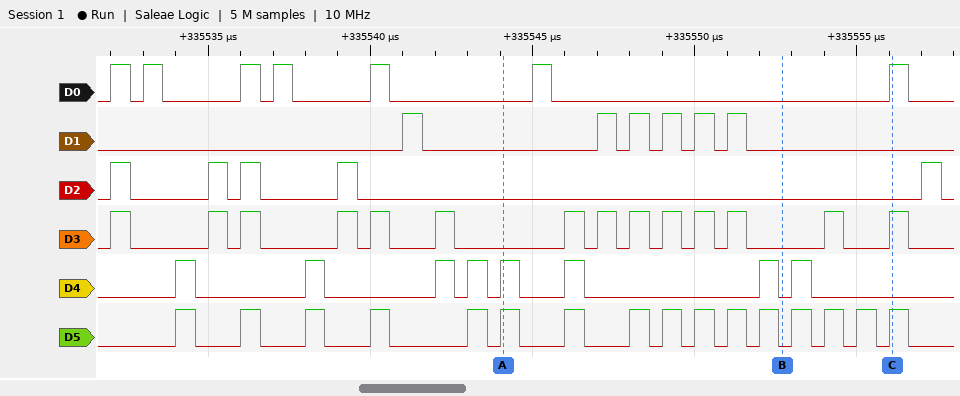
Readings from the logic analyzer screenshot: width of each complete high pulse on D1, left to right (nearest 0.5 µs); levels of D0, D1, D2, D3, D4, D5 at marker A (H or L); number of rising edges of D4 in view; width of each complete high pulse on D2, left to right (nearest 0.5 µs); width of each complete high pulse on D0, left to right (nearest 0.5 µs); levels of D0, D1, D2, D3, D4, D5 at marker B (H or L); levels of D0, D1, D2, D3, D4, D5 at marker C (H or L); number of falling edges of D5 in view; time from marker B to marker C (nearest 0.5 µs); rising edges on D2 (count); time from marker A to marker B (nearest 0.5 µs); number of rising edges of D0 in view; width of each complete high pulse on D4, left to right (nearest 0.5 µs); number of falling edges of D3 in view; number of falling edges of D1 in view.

0.5 µs, 0.5 µs, 0.5 µs, 0.5 µs, 0.5 µs, 0.5 µs
D0=L, D1=L, D2=L, D3=L, D4=H, D5=H
8
0.5 µs, 0.5 µs, 0.5 µs, 0.5 µs, 0.5 µs
0.5 µs, 0.5 µs, 0.5 µs, 0.5 µs, 0.5 µs, 0.5 µs, 0.5 µs
D0=L, D1=L, D2=L, D3=L, D4=L, D5=L
D0=H, D1=L, D2=L, D3=H, D4=L, D5=H
16
3.5 µs
5
8.5 µs
7
0.5 µs, 0.5 µs, 0.5 µs, 0.5 µs, 0.5 µs, 0.5 µs, 0.5 µs, 0.5 µs
14
6
